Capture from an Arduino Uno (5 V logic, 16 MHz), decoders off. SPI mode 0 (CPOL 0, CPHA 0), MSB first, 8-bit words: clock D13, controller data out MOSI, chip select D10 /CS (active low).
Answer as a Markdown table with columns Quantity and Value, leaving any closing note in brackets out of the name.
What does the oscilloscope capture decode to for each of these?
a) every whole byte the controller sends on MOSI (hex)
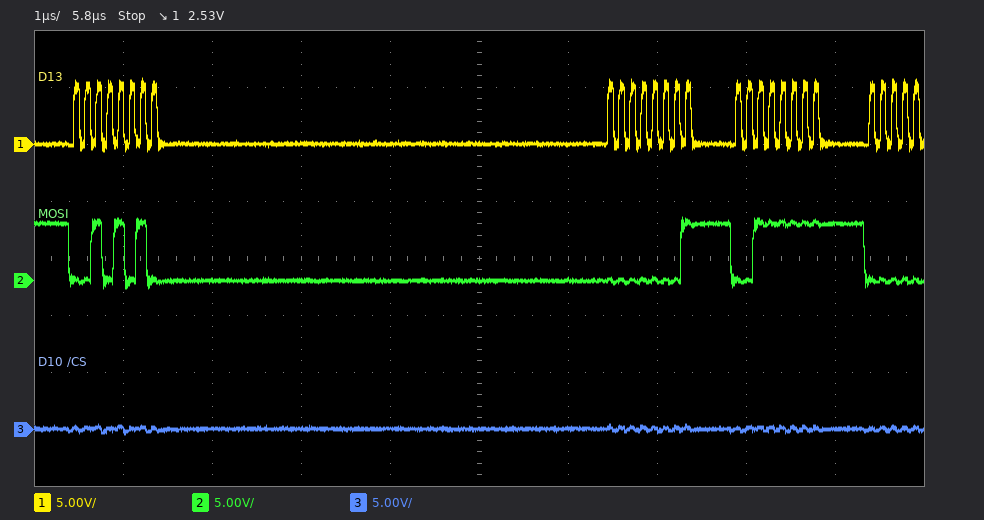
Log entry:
| Quantity | Value |
|---|---|
| every whole byte the controller sends on MOSI | 2A 01 3F |
